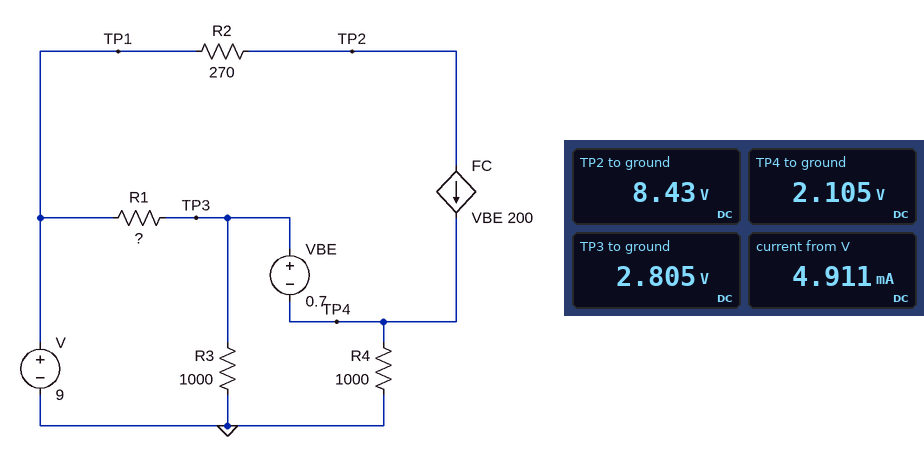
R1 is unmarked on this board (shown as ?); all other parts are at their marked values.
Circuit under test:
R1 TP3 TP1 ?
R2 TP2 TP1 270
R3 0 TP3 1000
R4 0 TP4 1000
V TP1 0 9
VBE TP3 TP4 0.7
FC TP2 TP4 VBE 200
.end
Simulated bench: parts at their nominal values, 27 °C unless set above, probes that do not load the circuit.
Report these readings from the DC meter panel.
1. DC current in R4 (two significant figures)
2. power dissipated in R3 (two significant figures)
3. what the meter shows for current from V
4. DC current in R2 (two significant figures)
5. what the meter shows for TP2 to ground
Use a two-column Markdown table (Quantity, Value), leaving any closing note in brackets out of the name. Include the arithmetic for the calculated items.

| Quantity | Value |
|---|---|
| DC current in R4 | (2.105 V) / 1 kΩ = 2.1 mA |
| power dissipated in R3 | (2.805 V)^2 / 1 kΩ = 7.9 mW |
| what the meter shows for current from V | 4.911 mA |
| DC current in R2 | (9 V - 8.43 V) / 270 Ω = 2.1 mA |
| what the meter shows for TP2 to ground | 8.43 V |
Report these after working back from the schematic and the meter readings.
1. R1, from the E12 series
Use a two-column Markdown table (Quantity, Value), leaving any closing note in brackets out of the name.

| Quantity | Value |
|---|---|
| R1, from the E12 series | 2.2 kΩ |
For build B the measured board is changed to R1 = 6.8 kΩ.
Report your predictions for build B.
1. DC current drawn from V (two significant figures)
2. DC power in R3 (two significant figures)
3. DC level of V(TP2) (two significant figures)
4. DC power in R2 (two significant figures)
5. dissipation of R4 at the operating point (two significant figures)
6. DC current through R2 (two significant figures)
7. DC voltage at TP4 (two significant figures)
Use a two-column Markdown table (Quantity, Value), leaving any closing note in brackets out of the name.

| Quantity | Value |
|---|---|
| DC current drawn from V | 1.6 mA |
| DC power in R3 | 1.3 mW |
| DC level of V(TP2) | 8.9 V |
| DC power in R2 | 55 µW |
| dissipation of R4 at the operating point | 200 µW |
| DC current through R2 | 450 µA |
| DC voltage at TP4 | 450 mV |
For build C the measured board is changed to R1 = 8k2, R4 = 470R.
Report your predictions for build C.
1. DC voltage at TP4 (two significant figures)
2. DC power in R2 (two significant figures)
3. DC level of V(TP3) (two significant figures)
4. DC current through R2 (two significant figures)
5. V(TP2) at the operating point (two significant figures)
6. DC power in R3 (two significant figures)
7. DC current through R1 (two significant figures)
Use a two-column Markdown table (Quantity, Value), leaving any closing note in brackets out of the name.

| Quantity | Value |
|---|---|
| DC voltage at TP4 | 280 mV |
| DC power in R2 | 92 µW |
| DC level of V(TP3) | 980 mV |
| DC current through R2 | 580 µA |
| V(TP2) at the operating point | 8.8 V |
| DC power in R3 | 950 µW |
| DC current through R1 | 980 µA |
